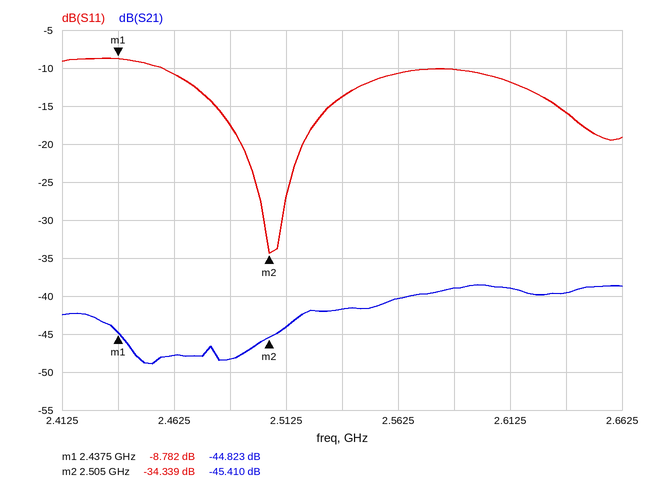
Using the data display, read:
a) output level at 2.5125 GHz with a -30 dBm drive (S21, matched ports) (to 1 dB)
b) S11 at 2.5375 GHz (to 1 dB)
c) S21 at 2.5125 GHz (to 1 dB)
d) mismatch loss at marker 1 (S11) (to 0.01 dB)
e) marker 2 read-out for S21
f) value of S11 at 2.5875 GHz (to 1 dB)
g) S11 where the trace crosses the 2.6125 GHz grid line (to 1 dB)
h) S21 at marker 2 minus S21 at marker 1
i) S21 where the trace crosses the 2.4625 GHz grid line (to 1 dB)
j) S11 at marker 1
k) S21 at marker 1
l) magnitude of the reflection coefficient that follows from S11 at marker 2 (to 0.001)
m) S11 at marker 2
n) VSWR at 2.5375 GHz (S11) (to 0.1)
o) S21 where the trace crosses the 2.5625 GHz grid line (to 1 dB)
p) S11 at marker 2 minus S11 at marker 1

-74 dBm
-14 dB
-44 dB
0.62 dB
-45.410 dB
-10 dB
-12 dB
-0.587 dB
-48 dB
-8.782 dB
-44.823 dB
0.019
-34.339 dB
1.5
-40 dB
-25.557 dB
